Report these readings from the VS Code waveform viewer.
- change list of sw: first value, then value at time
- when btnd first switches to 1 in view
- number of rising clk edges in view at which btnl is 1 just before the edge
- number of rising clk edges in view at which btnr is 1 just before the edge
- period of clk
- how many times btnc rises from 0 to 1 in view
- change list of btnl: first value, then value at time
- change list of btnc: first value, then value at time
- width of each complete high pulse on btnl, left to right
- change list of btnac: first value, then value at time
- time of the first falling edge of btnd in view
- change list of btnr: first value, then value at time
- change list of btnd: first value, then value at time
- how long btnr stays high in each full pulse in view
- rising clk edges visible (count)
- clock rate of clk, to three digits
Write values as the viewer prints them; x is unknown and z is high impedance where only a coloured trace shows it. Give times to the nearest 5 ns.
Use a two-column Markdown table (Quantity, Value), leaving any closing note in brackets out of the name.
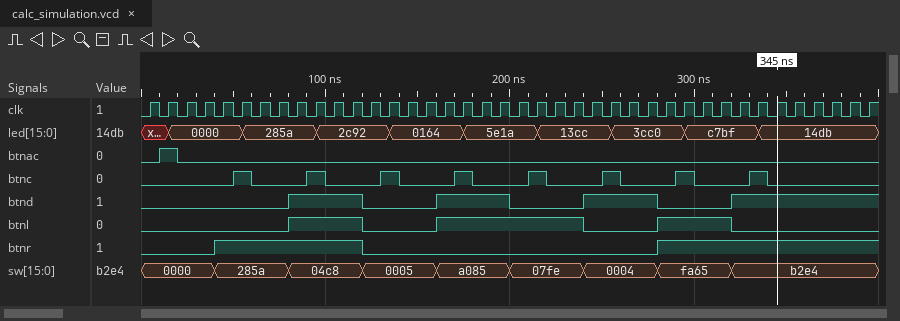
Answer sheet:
| Quantity | Value |
|---|---|
| change list of sw: first value, then value at time | 0000, 285a at 40 ns, 04c8 at 80 ns, 0005 at 120 ns, a085 at 160 ns, 07fe at 200 ns, 0004 at 240 ns, fa65 at 280 ns, b2e4 at 320 ns |
| when btnd first switches to 1 in view | 80 ns |
| number of rising clk edges in view at which btnl is 1 just before the edge | 16 |
| number of rising clk edges in view at which btnr is 1 just before the edge | 20 |
| period of clk | 10 ns |
| how many times btnc rises from 0 to 1 in view | 8 |
| change list of btnl: first value, then value at time | 0, 1 at 80 ns, 0 at 120 ns, 1 at 160 ns, 0 at 240 ns, 1 at 280 ns, 0 at 320 ns |
| change list of btnc: first value, then value at time | 0, 1 at 50 ns, 0 at 60 ns, 1 at 90 ns, 0 at 100 ns, 1 at 130 ns, 0 at 140 ns, 1 at 170 ns, 0 at 180 ns, 1 at 210 ns, 0 at 220 ns, 1 at 250 ns, 0 at 260 ns, 1 at 290 ns, 0 at 300 ns, 1 at 330 ns, 0 at 340 ns |
| width of each complete high pulse on btnl, left to right | 40 ns, 80 ns, 40 ns |
| change list of btnac: first value, then value at time | 0, 1 at 10 ns, 0 at 20 ns |
| time of the first falling edge of btnd in view | 120 ns |
| change list of btnr: first value, then value at time | 0, 1 at 40 ns, 0 at 120 ns, 1 at 280 ns |
| change list of btnd: first value, then value at time | 0, 1 at 80 ns, 0 at 120 ns, 1 at 160 ns, 0 at 200 ns, 1 at 240 ns, 0 at 280 ns, 1 at 320 ns |
| how long btnr stays high in each full pulse in view | 80 ns |
| rising clk edges visible | 40 |
| clock rate of clk, to three digits | 100 MHz |
